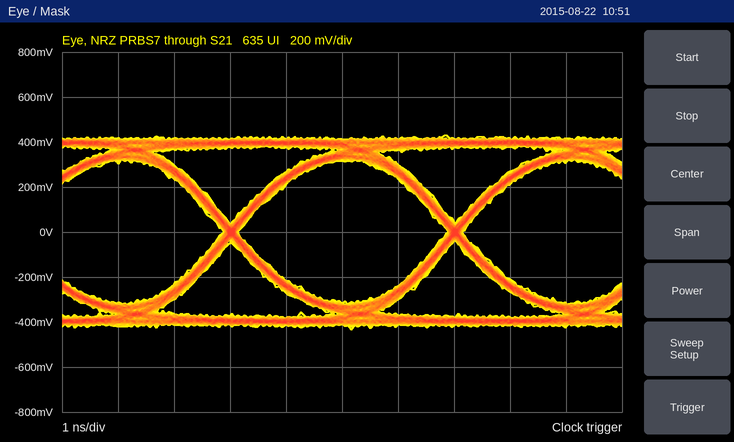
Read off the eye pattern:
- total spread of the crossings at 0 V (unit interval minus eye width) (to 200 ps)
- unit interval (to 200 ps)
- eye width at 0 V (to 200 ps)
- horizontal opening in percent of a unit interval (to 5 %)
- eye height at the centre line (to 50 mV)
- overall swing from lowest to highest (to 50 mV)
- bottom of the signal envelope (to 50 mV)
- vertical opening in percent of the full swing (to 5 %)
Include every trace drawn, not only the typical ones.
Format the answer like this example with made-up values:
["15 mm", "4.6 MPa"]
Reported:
["200 ps", "4.0 ns", "3.8 ns", "95 %", "650 mV", "850 mV", "-450 mV", "75 %"]
